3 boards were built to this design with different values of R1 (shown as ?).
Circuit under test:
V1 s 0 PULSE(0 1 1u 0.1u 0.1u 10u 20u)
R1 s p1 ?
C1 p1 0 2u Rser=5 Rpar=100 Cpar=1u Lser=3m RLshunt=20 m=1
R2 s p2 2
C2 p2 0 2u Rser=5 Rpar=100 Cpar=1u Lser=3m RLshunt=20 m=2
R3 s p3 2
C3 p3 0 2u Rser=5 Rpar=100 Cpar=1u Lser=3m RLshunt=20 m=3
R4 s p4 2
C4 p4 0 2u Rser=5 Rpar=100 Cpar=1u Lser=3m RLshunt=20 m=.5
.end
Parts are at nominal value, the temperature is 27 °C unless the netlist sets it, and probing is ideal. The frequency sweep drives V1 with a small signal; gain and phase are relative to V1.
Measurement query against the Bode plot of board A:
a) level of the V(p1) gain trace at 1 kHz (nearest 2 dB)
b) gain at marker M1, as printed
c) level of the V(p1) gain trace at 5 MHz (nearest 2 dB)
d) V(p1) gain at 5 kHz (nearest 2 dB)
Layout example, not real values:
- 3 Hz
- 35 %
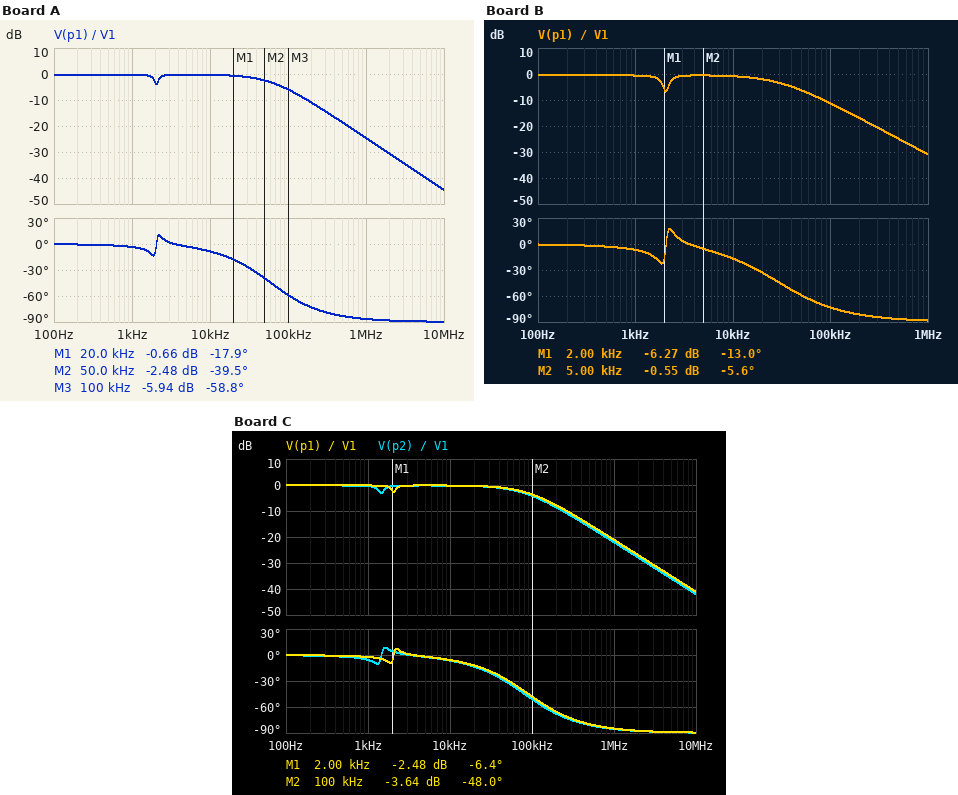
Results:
- 0 dB
- -0.66 dB
- -38 dB
- 0 dB
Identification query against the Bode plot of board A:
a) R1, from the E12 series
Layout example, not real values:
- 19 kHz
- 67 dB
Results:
- 2.7 Ω
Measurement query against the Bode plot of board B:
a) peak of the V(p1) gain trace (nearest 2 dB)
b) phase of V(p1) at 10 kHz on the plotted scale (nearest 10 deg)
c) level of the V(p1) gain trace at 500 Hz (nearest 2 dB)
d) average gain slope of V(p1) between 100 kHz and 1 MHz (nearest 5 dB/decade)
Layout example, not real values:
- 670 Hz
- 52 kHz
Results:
- 0 dB
- -20 deg
- 0 dB
- -20 dB/decade
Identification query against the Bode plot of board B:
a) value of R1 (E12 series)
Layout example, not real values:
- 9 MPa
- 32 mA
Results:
- 5.6 Ω
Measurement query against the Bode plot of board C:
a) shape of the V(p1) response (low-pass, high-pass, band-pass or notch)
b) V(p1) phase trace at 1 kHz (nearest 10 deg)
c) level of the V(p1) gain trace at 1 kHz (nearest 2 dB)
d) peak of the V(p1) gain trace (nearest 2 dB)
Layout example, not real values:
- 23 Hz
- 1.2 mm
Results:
- low-pass
- 0 deg
- 0 dB
- 0 dB
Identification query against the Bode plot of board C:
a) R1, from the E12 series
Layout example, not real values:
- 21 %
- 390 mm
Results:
- 1.8 Ω
